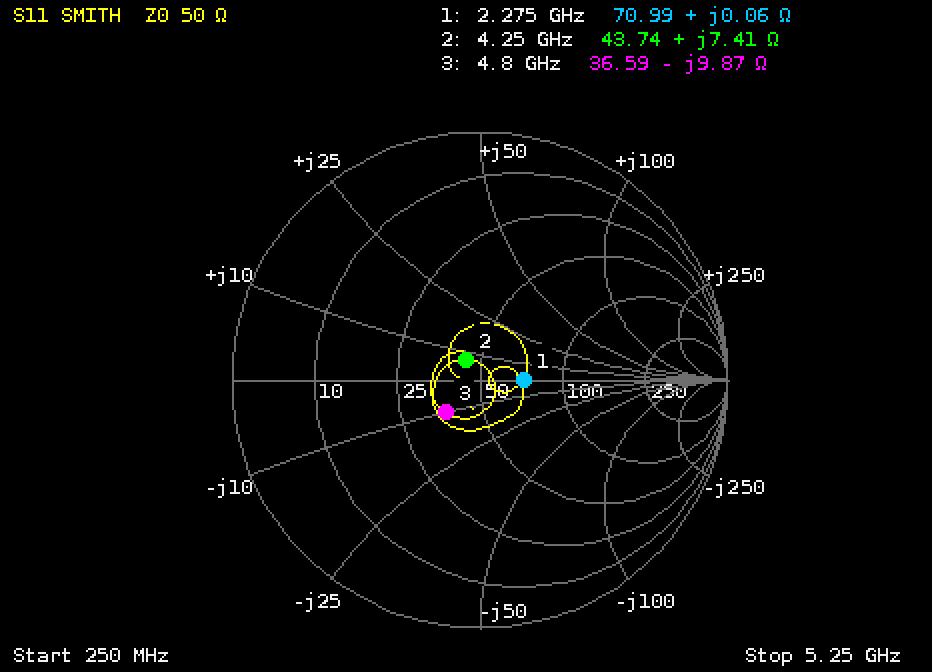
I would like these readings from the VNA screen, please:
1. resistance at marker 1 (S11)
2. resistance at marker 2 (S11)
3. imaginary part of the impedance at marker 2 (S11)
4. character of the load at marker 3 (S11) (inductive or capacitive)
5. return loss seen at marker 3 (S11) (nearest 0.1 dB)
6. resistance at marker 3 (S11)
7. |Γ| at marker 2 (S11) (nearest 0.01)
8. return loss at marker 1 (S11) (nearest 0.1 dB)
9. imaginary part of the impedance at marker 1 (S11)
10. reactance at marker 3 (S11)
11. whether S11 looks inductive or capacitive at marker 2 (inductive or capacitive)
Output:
70.99 Ω
43.74 Ω
+7.41 Ω
capacitive
14.4 dB
36.59 Ω
0.10
15.2 dB
+0.06 Ω
-9.87 Ω
inductive
